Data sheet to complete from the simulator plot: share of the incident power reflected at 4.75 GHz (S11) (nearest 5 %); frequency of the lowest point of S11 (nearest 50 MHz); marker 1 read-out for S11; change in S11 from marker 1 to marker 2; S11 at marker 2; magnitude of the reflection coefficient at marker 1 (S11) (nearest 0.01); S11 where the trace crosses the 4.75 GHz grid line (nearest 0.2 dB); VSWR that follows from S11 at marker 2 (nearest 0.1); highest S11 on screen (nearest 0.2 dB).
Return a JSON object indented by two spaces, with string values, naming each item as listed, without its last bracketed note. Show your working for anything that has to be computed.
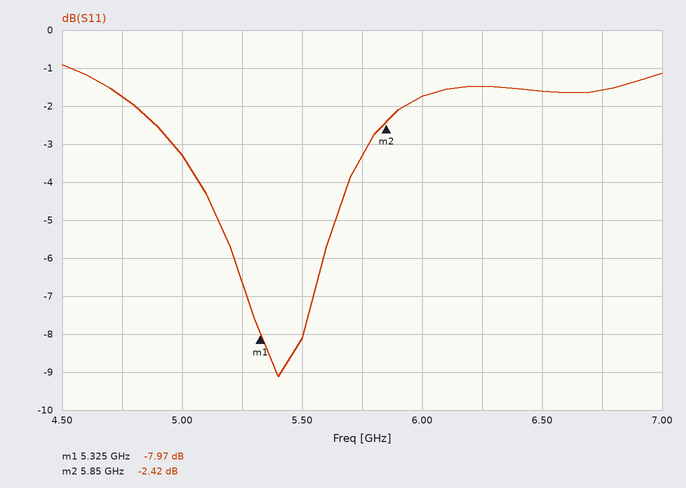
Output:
{
  "share of the incident power reflected at 4.75 GHz (S11)": "10^(-1.8/10) ≈ 66.1 %, so 65 % to the nearest 5 %",
  "frequency of the lowest point of S11": "5.40 GHz",
  "marker 1 read-out for S11": "-7.97 dB",
  "change in S11 from marker 1 to marker 2": "-2.42 − (-7.97) = 5.55 dB",
  "S11 at marker 2": "-2.42 dB",
  "magnitude of the reflection coefficient at marker 1 (S11)": "10^(-7.97/20) ≈ 0.40",
  "S11 where the trace crosses the 4.75 GHz grid line": "-1.8 dB",
  "VSWR that follows from S11 at marker 2": "(1 + 0.7568)/(1 − 0.7568) ≈ 7.2",
  "highest S11 on screen": "-1.0 dB"
}
